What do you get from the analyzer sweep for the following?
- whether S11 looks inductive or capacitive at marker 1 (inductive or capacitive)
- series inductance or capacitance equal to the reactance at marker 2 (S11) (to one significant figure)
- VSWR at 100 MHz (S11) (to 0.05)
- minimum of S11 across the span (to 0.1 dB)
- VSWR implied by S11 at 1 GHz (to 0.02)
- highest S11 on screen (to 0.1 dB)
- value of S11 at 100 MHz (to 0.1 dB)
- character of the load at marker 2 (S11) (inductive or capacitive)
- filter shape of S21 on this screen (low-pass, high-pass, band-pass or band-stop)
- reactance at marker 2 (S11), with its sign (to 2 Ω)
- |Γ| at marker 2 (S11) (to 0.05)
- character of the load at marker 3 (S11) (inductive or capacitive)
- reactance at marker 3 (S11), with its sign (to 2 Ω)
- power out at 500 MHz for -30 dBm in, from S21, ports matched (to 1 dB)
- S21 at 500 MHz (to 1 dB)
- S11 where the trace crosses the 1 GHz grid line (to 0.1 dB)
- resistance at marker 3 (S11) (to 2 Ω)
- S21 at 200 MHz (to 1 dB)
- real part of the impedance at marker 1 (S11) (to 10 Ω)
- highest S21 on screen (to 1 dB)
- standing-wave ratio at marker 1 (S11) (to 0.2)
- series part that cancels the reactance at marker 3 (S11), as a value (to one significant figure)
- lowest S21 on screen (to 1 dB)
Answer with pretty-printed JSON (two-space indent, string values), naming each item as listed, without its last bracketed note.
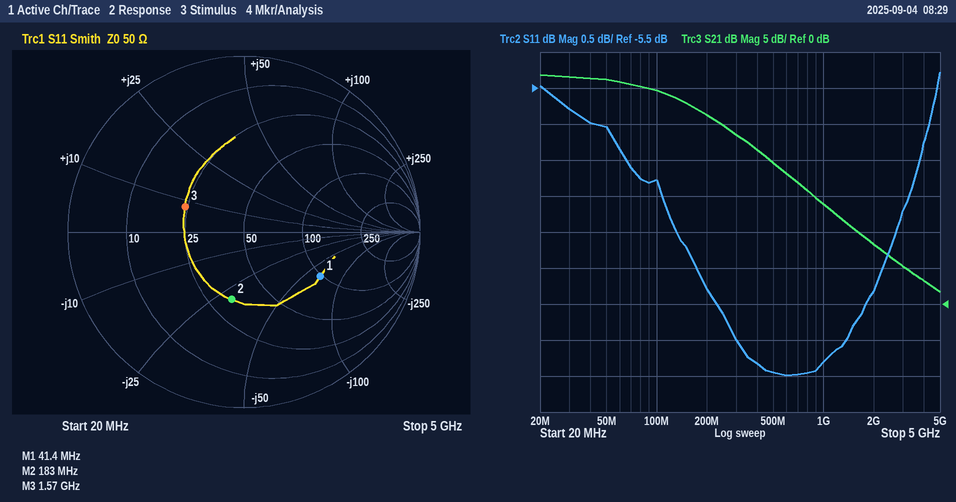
{
  "whether S11 looks inductive or capacitive at marker 1": "capacitive",
  "series inductance or capacitance equal to the reactance at marker 2 (S11)": "30 pF",
  "VSWR at 100 MHz (S11)": "2.70",
  "minimum of S11 across the span": "-9.5 dB",
  "VSWR implied by S11 at 1 GHz": "2.04",
  "highest S11 on screen": "-5.3 dB",
  "value of S11 at 100 MHz": "-6.8 dB",
  "character of the load at marker 2 (S11)": "capacitive",
  "filter shape of S21 on this screen": "low-pass",
  "reactance at marker 2 (S11), with its sign": "-30 Ω",
  "|Γ| at marker 2 (S11)": "0.40",
  "character of the load at marker 3 (S11)": "inductive",
  "reactance at marker 3 (S11), with its sign": "+8 Ω",
  "power out at 500 MHz for -30 dBm in, from S21, ports matched": "-10 dBm",
  "S21 at 500 MHz": "20 dB",
  "S11 where the trace crosses the 1 GHz grid line": "-9.3 dB",
  "resistance at marker 3 (S11)": "24 Ω",
  "S21 at 200 MHz": "26 dB",
  "real part of the impedance at marker 1 (S11)": "100 Ω",
  "highest S21 on screen": "32 dB",
  "standing-wave ratio at marker 1 (S11)": "3.0",
  "series part that cancels the reactance at marker 3 (S11), as a value": "10 pF",
  "lowest S21 on screen": "2 dB"
}
